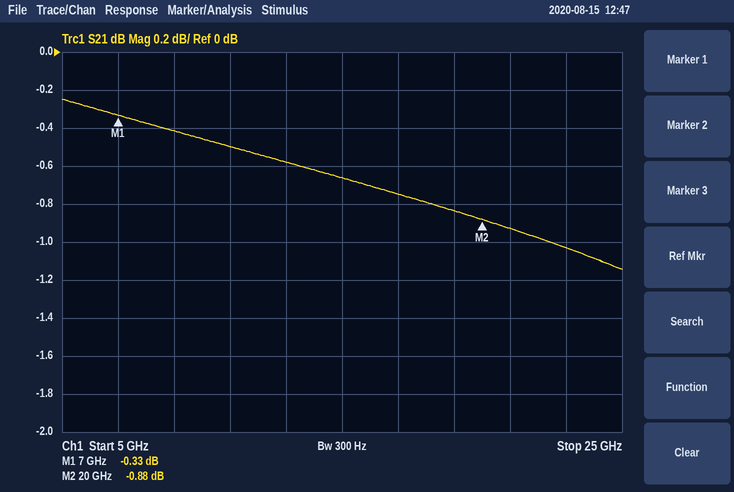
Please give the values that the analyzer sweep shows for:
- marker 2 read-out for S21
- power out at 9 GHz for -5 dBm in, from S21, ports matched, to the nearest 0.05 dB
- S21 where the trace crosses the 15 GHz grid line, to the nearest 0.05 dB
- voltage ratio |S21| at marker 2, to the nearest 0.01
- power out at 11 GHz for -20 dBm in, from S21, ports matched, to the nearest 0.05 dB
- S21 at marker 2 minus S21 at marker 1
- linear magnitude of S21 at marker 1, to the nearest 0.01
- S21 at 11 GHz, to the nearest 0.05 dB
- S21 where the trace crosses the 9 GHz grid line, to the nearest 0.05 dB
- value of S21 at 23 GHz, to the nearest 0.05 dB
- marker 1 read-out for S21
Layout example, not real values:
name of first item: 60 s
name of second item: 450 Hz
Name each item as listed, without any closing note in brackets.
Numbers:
marker 2 read-out for S21: -0.88 dB
power out at 9 GHz for -5 dBm in, from S21, ports matched, to the nearest 0.05 dB: -5.40 dBm
S21 where the trace crosses the 15 GHz grid line, to the nearest 0.05 dB: -0.65 dB
voltage ratio |S21| at marker 2, to the nearest 0.01: 0.90
power out at 11 GHz for -20 dBm in, from S21, ports matched, to the nearest 0.05 dB: -20.50 dBm
S21 at marker 2 minus S21 at marker 1: -0.55 dB
linear magnitude of S21 at marker 1, to the nearest 0.01: 0.96
S21 at 11 GHz, to the nearest 0.05 dB: -0.50 dB
S21 where the trace crosses the 9 GHz grid line, to the nearest 0.05 dB: -0.40 dB
value of S21 at 23 GHz, to the nearest 0.05 dB: -1.05 dB
marker 1 read-out for S21: -0.33 dB
